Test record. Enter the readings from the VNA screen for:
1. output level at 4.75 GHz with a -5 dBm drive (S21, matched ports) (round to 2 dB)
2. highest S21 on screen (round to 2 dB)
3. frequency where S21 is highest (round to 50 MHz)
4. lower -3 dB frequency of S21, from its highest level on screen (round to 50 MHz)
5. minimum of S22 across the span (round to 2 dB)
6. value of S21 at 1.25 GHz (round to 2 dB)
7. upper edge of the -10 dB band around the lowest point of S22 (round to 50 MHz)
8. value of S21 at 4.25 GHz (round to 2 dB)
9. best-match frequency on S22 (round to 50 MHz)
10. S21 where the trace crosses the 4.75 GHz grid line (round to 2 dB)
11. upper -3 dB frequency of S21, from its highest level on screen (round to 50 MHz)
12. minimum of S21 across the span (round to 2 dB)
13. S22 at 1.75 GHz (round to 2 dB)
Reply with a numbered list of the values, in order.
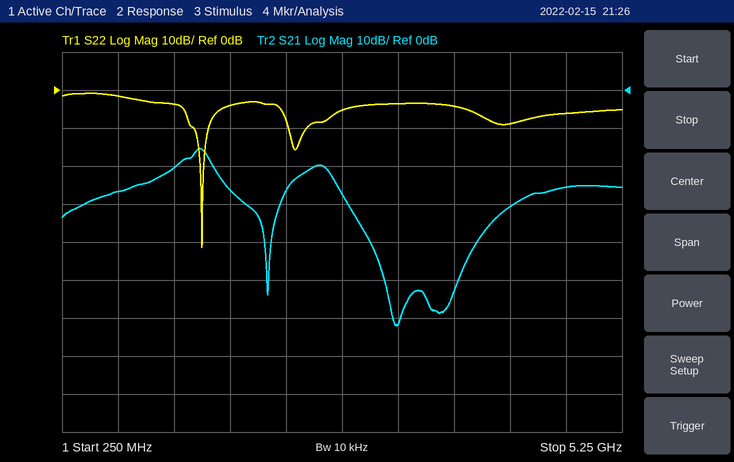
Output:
1. -30 dBm
2. -16 dB
3. 1.50 GHz
4. 1.35 GHz
5. -42 dB
6. -20 dB
7. 1.55 GHz
8. -30 dB
9. 1.50 GHz
10. -26 dB
11. 1.55 GHz
12. -62 dB
13. -4 dB
